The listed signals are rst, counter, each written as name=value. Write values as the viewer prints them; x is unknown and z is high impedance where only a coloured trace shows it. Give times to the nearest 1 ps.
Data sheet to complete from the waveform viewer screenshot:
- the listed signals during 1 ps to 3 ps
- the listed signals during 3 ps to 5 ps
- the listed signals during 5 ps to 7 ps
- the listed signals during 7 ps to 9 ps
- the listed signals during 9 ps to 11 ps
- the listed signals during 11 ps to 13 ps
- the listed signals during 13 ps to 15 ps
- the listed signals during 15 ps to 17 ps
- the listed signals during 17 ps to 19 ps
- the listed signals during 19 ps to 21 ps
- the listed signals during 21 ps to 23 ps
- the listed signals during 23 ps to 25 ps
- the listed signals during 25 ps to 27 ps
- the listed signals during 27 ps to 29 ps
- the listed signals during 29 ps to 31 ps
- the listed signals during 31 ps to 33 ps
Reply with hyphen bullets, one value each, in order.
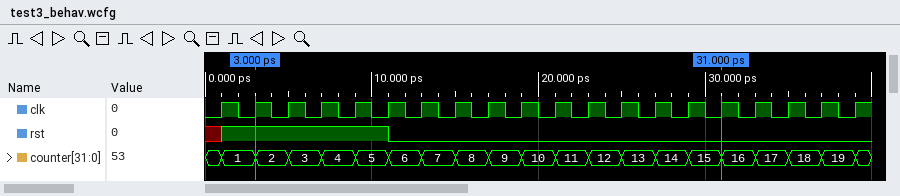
- rst=1, counter=1
- rst=1, counter=2
- rst=1, counter=3
- rst=1, counter=4
- rst=1, counter=5
- rst=0, counter=6
- rst=0, counter=7
- rst=0, counter=8
- rst=0, counter=9
- rst=0, counter=10
- rst=0, counter=11
- rst=0, counter=12
- rst=0, counter=13
- rst=0, counter=14
- rst=0, counter=15
- rst=0, counter=16
